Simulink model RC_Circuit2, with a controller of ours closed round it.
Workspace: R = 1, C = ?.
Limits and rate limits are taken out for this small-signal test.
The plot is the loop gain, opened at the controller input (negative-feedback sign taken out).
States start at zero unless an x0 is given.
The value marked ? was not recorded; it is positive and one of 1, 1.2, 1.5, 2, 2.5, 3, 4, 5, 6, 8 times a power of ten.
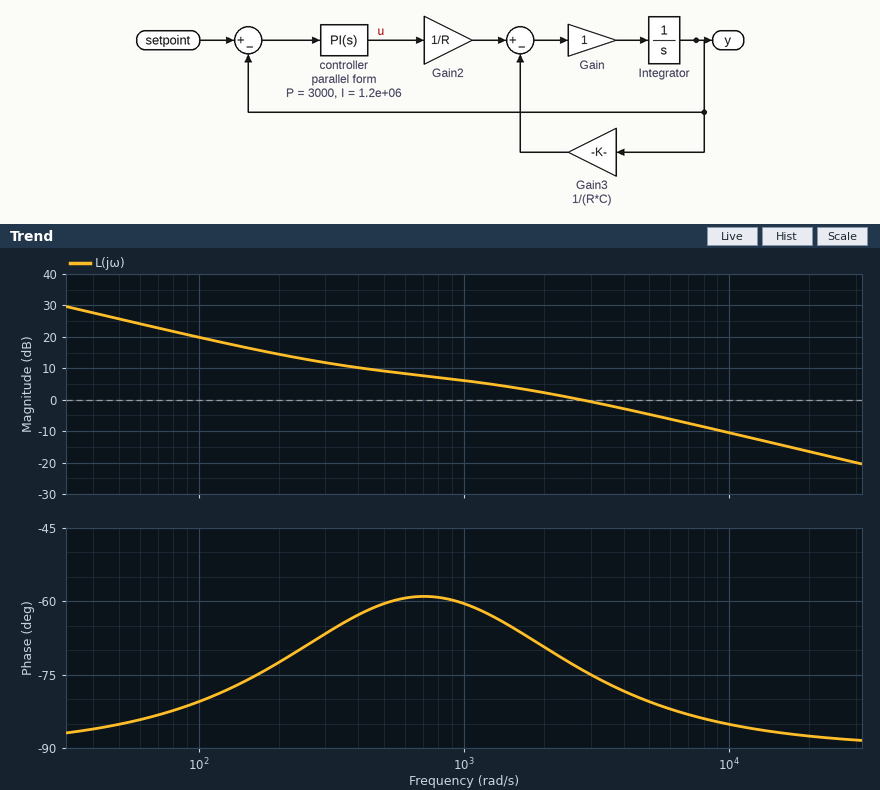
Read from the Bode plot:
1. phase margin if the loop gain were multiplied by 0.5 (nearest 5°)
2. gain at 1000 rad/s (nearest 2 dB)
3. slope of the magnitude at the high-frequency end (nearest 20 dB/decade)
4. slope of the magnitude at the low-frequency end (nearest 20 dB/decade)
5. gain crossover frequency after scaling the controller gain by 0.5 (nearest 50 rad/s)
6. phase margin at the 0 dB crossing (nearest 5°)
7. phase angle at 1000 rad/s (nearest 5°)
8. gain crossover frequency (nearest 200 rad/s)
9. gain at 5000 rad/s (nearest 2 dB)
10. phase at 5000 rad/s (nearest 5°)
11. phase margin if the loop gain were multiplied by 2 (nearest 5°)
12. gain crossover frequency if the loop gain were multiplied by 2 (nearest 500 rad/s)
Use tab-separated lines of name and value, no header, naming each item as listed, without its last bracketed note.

phase margin if the loop gain were multiplied by 0.5	120°
gain at 1000 rad/s	6 dB
slope of the magnitude at the high-frequency end	-20 dB/decade
slope of the magnitude at the low-frequency end	-20 dB/decade
gain crossover frequency after scaling the controller gain by 0.5	1000 rad/s
phase margin at the 0 dB crossing	105°
phase angle at 1000 rad/s	-60°
gain crossover frequency	2800 rad/s
gain at 5000 rad/s	-4 dB
phase at 5000 rad/s	-80°
phase margin if the loop gain were multiplied by 2	100°
gain crossover frequency if the loop gain were multiplied by 2	6000 rad/s
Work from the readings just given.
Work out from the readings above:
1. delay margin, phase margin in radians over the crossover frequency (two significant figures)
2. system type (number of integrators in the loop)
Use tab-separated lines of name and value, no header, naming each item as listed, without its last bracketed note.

delay margin, phase margin in radians over the crossover frequency	0.00065 s
system type	1
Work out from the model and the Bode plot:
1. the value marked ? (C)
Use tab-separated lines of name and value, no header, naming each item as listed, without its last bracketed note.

the value marked ?	0.0008
